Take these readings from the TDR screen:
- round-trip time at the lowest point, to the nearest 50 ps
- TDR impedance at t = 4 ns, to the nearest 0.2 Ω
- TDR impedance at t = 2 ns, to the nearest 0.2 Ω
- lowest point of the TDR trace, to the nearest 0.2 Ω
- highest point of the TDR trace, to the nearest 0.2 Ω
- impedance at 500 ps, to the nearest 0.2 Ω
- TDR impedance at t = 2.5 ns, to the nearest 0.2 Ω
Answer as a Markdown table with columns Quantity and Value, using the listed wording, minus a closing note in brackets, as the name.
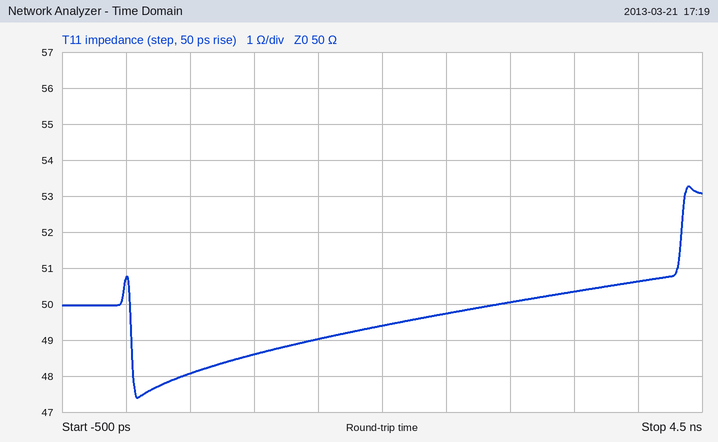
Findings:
| Quantity | Value |
|---|---|
| round-trip time at the lowest point, to the nearest 50 ps | 100 ps |
| TDR impedance at t = 4 ns, to the nearest 0.2 Ω | 50.6 Ω |
| TDR impedance at t = 2 ns, to the nearest 0.2 Ω | 49.4 Ω |
| lowest point of the TDR trace, to the nearest 0.2 Ω | 47.4 Ω |
| highest point of the TDR trace, to the nearest 0.2 Ω | 53.2 Ω |
| impedance at 500 ps, to the nearest 0.2 Ω | 48.0 Ω |
| TDR impedance at t = 2.5 ns, to the nearest 0.2 Ω | 49.8 Ω |
